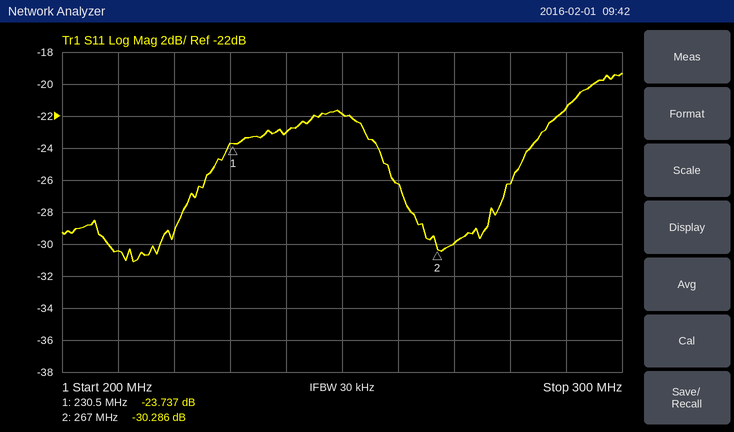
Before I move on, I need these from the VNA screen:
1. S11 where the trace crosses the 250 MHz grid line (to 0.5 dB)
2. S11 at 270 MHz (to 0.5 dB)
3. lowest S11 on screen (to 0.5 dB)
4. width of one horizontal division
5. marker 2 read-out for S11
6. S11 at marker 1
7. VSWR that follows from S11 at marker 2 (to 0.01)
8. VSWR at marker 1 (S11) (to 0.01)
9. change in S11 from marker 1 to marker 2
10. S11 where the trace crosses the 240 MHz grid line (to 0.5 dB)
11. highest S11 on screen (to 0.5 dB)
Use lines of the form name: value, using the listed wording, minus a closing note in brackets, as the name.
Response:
S11 where the trace crosses the 250 MHz grid line: -22.0 dB
S11 at 270 MHz: -30.0 dB
lowest S11 on screen: -31.0 dB
width of one horizontal division: 10 MHz
marker 2 read-out for S11: -30.286 dB
S11 at marker 1: -23.737 dB
VSWR that follows from S11 at marker 2: 1.06
VSWR at marker 1 (S11): 1.14
change in S11 from marker 1 to marker 2: -6.549 dB
S11 where the trace crosses the 240 MHz grid line: -23.0 dB
highest S11 on screen: -19.5 dB
